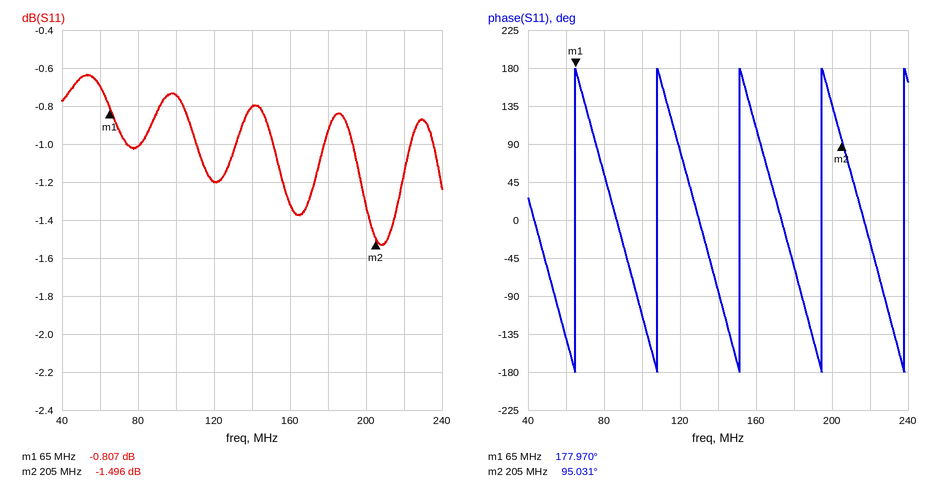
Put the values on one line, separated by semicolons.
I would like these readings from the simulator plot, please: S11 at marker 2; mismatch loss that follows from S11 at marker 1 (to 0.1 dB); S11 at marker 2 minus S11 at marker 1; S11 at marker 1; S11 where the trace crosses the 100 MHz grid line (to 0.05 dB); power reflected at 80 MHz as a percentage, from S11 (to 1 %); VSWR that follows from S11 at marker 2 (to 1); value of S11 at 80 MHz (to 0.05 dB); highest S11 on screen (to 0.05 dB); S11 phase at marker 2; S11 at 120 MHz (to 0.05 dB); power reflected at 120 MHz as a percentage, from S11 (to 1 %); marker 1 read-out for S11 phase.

-1.496 dB; 7.7 dB; -0.689 dB; -0.807 dB; -0.75 dB; 79 %; 12; -1.00 dB; -0.65 dB; 95.031°; -1.20 dB; 76 %; 177.970°
